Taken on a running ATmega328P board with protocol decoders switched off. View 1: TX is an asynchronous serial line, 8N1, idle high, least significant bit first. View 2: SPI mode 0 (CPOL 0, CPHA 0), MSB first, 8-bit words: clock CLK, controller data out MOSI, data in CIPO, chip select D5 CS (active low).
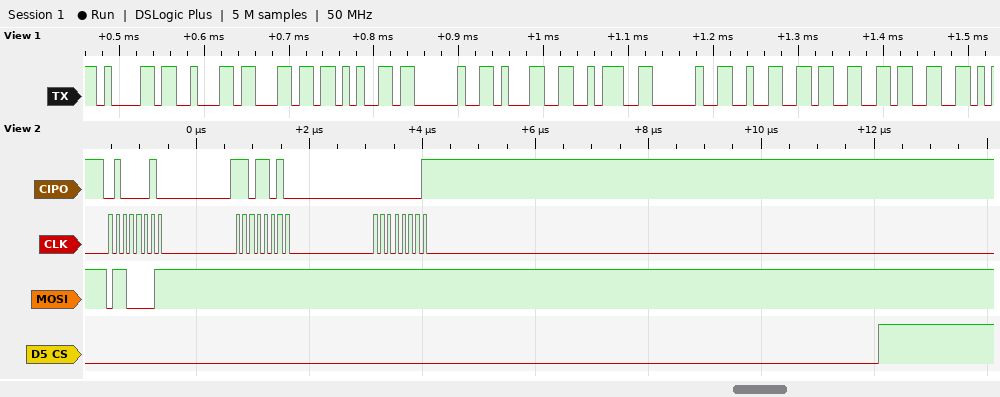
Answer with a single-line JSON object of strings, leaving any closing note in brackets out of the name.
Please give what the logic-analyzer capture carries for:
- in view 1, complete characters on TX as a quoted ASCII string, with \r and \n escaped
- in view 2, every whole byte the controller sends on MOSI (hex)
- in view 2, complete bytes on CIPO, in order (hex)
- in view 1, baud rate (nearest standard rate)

{"in view 1, complete characters on TX as a quoted ASCII string, with \\r and \\n escaped": "\"able 1: 233\"", "in view 2, every whole byte the controller sends on MOSI": "61 FF FF", "in view 2, complete bytes on CIPO, in order": "42 DA 01", "in view 1, baud rate": "115200 baud"}
